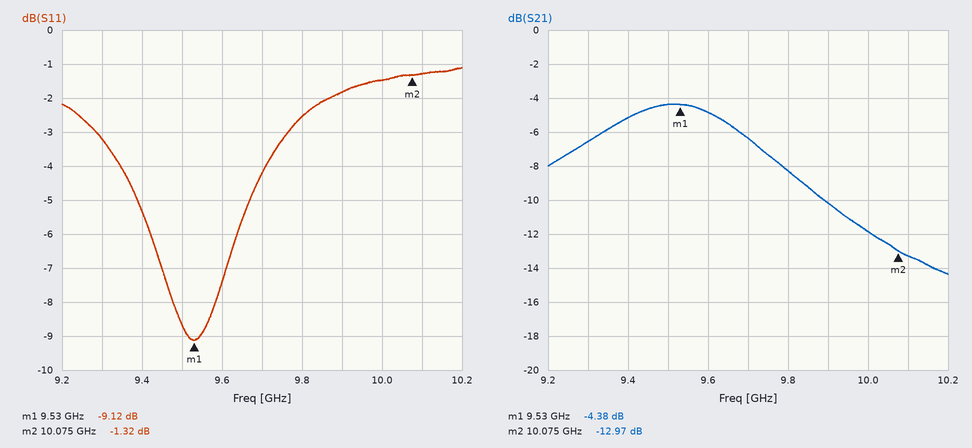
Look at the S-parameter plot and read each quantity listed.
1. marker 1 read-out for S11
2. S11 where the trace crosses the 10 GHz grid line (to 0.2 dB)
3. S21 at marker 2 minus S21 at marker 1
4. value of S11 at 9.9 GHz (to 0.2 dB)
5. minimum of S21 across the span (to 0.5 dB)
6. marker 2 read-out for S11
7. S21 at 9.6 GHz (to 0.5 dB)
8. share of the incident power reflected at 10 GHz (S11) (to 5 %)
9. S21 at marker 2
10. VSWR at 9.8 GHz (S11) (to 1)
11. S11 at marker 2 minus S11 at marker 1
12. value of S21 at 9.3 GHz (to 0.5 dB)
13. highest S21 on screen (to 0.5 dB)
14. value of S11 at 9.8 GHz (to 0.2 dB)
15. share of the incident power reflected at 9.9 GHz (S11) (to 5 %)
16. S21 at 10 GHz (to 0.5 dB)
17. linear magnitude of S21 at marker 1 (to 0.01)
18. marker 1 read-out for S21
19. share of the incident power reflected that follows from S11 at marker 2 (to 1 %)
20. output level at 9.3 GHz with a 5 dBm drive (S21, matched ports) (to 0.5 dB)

-9.12 dB
-1.4 dB
-8.59 dB
-1.8 dB
-14.5 dB
-1.32 dB
-5.0 dB
70 %
-12.97 dB
7
7.80 dB
-6.5 dB
-4.5 dB
-2.6 dB
65 %
-12.0 dB
0.60
-4.38 dB
74 %
-1.5 dBm
